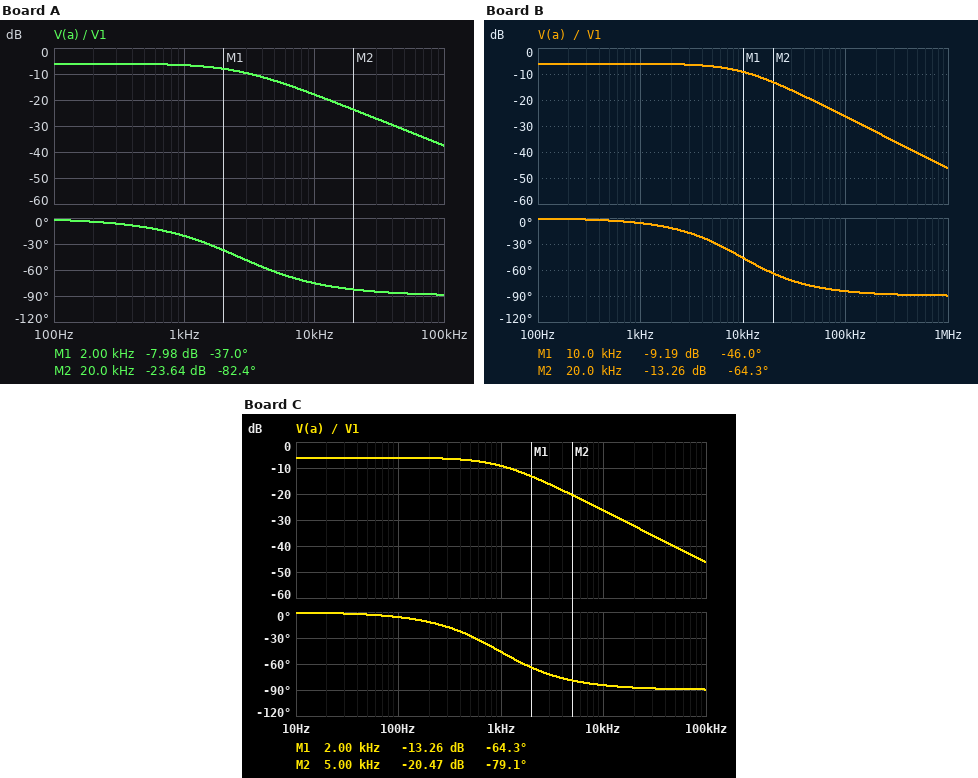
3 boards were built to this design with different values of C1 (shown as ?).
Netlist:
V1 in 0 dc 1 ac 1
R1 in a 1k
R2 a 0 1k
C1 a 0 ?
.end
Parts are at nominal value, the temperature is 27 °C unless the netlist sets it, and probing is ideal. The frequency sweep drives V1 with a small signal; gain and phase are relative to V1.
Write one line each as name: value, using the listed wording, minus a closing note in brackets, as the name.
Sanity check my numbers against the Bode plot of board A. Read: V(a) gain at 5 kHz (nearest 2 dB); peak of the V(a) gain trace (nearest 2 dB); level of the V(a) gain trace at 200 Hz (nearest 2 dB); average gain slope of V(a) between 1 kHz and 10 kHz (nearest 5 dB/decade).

V(a) gain at 5 kHz: -12 dB
peak of the V(a) gain trace: -6 dB
level of the V(a) gain trace at 200 Hz: -6 dB
average gain slope of V(a) between 1 kHz and 10 kHz: -10 dB/decade
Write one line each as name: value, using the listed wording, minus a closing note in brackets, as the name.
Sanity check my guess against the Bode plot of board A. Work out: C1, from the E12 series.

C1, from the E12 series: 120 nF
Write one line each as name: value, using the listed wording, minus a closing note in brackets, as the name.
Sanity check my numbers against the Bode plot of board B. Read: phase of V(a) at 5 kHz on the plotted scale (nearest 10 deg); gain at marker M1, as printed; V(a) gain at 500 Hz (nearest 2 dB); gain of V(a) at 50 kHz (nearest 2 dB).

phase of V(a) at 5 kHz on the plotted scale: -30 deg
gain at marker M1, as printed: -9.19 dB
V(a) gain at 500 Hz: -6 dB
gain of V(a) at 50 kHz: -20 dB
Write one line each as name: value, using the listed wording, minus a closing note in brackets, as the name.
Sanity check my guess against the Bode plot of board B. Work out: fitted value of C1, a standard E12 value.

fitted value of C1, a standard E12 value: 33 nF
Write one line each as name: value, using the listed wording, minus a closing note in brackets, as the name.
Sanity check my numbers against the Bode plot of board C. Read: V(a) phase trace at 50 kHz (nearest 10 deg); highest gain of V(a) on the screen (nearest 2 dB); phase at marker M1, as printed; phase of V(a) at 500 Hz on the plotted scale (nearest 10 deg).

V(a) phase trace at 50 kHz: -90 deg
highest gain of V(a) on the screen: -6 dB
phase at marker M1, as printed: -64.3 deg
phase of V(a) at 500 Hz on the plotted scale: -30 deg
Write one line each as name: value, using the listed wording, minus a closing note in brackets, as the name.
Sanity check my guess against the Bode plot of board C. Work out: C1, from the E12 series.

C1, from the E12 series: 330 nF
